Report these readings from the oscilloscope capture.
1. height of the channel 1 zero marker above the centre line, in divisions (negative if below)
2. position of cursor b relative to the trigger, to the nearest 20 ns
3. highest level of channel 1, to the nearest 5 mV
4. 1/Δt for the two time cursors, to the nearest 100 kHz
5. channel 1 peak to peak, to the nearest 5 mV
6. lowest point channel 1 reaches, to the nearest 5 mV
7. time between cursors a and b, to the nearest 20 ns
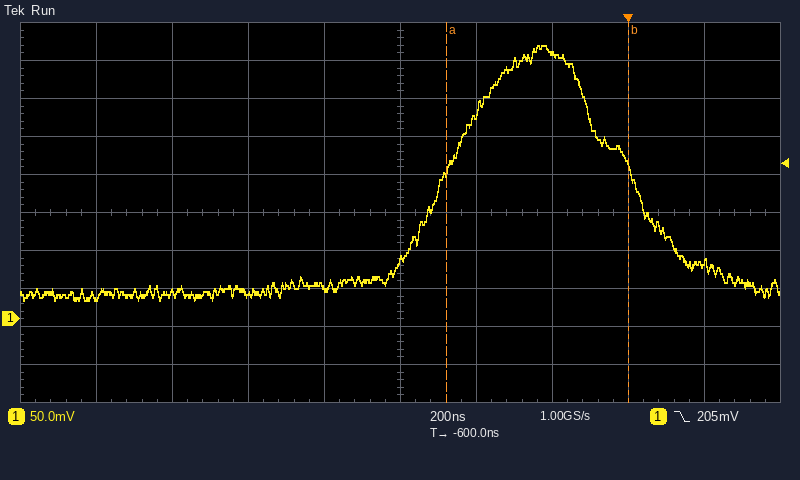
-2.8 div
0 ns
360 mV
2.1 MHz
335 mV
25 mV
480 ns
